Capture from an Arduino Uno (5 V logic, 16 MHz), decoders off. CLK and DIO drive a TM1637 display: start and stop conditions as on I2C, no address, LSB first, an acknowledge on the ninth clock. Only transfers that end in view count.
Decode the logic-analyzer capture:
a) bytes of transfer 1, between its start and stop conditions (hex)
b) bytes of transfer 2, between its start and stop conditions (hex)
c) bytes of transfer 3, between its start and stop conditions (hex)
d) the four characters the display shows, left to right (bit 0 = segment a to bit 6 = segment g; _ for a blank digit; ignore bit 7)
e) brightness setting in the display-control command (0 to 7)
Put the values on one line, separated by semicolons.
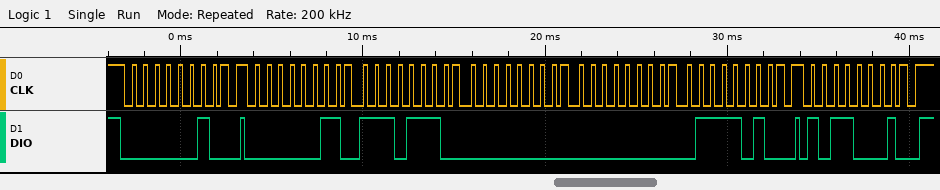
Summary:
40; C0 77 00 00 5E; 8D; A__d; 5
